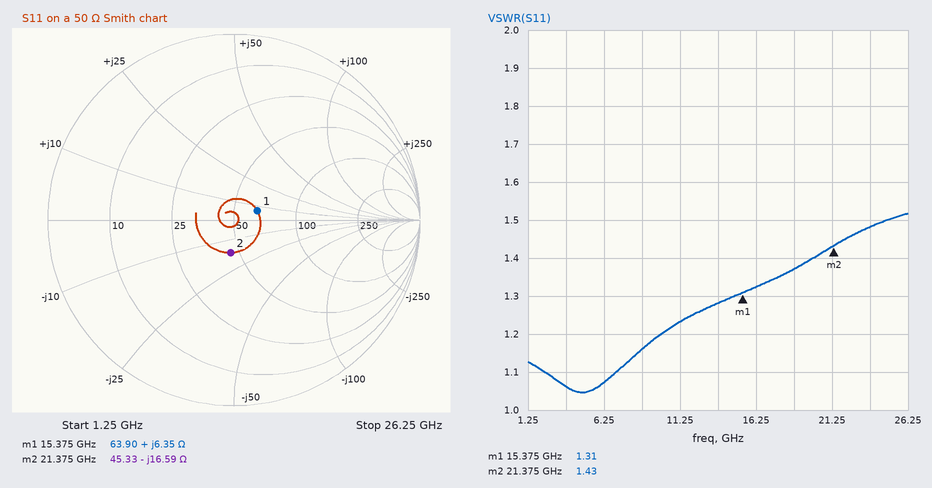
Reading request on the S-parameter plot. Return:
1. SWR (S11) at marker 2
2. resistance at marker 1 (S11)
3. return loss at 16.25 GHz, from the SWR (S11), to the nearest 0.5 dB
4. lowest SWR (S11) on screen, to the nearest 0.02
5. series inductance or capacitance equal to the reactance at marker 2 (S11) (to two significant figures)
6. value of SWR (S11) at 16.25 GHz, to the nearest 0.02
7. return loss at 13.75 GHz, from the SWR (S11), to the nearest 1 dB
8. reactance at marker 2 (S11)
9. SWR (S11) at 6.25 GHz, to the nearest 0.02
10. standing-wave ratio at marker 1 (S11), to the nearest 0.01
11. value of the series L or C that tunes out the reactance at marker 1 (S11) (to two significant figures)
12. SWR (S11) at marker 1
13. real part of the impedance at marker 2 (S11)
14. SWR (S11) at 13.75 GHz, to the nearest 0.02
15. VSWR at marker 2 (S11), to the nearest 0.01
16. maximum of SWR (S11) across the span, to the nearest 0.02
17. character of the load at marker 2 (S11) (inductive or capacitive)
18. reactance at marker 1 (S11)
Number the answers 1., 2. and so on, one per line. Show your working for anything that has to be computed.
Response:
1. 1.43
2. 63.90 Ω
3. −20 log10((1.32 − 1)/(1.32 + 1)) ≈ 17.2 dB, so 17.0 dB to the nearest 0.5 dB
4. 1.04
5. C = 1/(2π × 21.375 GHz × 16.59 Ω) ≈ 449 fF, so 450 fF to two significant figures
6. 1.32
7. −20 log10((1.28 − 1)/(1.28 + 1)) ≈ 18 dB
8. -16.59 Ω
9. 1.08
10. 1.31
11. C = 1/(2π × 15.375 GHz × 6.35 Ω) ≈ 1.6 pF
12. 1.31
13. 45.33 Ω
14. 1.28
15. 1.43
16. 1.52
17. capacitive
18. +6.35 Ω
